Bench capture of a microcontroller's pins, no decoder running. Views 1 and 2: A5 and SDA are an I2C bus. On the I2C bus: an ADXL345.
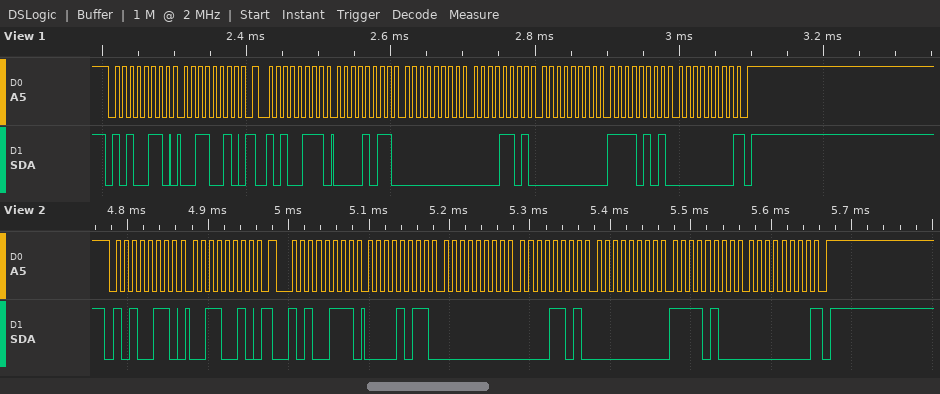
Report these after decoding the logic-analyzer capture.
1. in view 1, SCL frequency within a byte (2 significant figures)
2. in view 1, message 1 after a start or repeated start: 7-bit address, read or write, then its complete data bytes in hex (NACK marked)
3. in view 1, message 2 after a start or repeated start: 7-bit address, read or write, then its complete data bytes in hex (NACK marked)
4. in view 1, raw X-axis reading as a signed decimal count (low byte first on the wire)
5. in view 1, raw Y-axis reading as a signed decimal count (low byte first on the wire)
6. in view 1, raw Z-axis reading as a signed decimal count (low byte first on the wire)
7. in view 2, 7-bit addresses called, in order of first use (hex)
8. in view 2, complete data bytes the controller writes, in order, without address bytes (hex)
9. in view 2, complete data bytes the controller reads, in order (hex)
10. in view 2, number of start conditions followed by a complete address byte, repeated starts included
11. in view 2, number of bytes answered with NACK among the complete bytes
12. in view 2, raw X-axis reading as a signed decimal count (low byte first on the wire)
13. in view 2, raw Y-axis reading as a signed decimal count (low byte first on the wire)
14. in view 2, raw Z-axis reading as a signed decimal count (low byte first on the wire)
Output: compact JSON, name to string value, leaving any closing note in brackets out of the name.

{"in view 1, SCL frequency within a byte": "100 kHz", "in view 1, message 1 after a start or repeated start: 7-bit address, read or write, then its complete data bytes in hex": "0x53 write: 32", "in view 1, message 2 after a start or repeated start: 7-bit address, read or write, then its complete data bytes in hex": "0x53 read: 0B 00 0D 00 F5 00 NACK", "in view 1, raw X-axis reading as a signed decimal count": "11", "in view 1, raw Y-axis reading as a signed decimal count": "13", "in view 1, raw Z-axis reading as a signed decimal count": "245", "in view 2, 7-bit addresses called, in order of first use": "0x53", "in view 2, complete data bytes the controller writes, in order, without address bytes": "32", "in view 2, complete data bytes the controller reads, in order": "0B 00 0D 00 F4 00", "in view 2, number of start conditions followed by a complete address byte, repeated starts included": "2", "in view 2, number of bytes answered with NACK among the complete bytes": "1", "in view 2, raw X-axis reading as a signed decimal count": "11", "in view 2, raw Y-axis reading as a signed decimal count": "13", "in view 2, raw Z-axis reading as a signed decimal count": "244"}
